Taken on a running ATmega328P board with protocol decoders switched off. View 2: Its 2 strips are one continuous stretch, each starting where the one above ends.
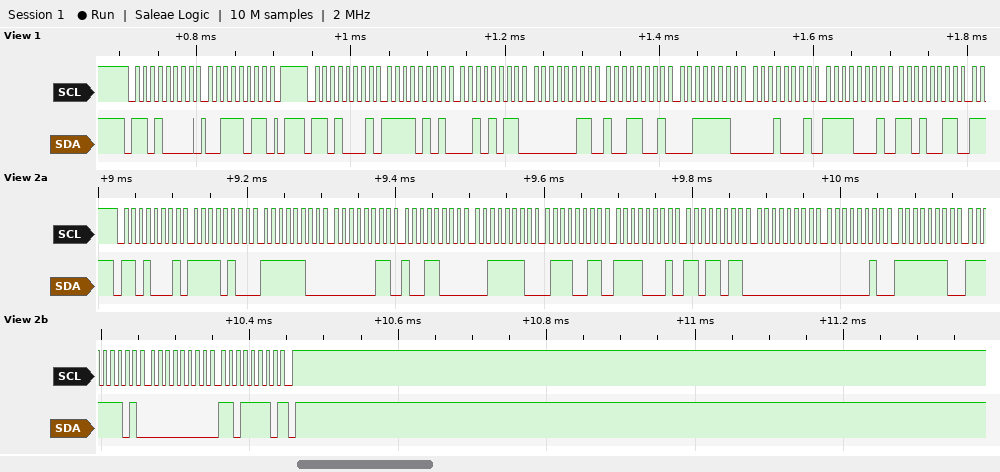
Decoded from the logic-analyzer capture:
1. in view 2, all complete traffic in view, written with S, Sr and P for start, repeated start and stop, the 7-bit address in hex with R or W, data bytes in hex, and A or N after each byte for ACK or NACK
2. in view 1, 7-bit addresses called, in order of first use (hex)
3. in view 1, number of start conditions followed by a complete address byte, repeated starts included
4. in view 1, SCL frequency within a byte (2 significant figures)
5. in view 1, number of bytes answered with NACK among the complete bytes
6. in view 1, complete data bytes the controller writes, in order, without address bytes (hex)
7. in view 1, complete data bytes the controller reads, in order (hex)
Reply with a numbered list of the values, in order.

1. S 68R A F4 A FC A 03 A 98 A 3E A 73 A F1 A DB A 00 A 02 A FE A FD A 00 A DE N P
2. 0x68
3. 2
4. 100 kHz
5. 0
6. 3B
7. F5 2B 03 99 3E 11 F1 D3
